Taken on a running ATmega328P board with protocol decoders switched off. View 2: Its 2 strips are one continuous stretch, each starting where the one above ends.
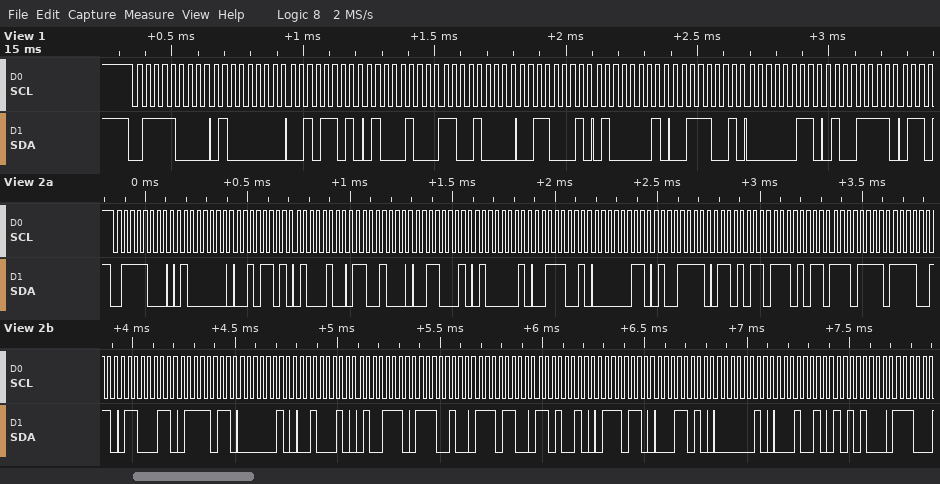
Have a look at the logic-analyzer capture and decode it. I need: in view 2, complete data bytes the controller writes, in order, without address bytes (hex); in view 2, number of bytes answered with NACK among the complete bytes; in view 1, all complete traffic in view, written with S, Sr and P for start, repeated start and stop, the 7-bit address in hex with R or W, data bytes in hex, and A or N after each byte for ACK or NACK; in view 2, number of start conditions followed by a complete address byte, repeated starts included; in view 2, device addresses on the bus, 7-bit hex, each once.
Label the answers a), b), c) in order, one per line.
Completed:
a) 40 2D 44 C8 31 41 39 03 4F 6B EB EF F3 63 7B 02 22 4E E4 EC D2 76 1A 02 12 A8
b) 0
c) S 3CW A 40 A 2D A 44 A C8 A 31 A 41 A 39 A 03 A 4F A
d) 1
e) 0x3C
